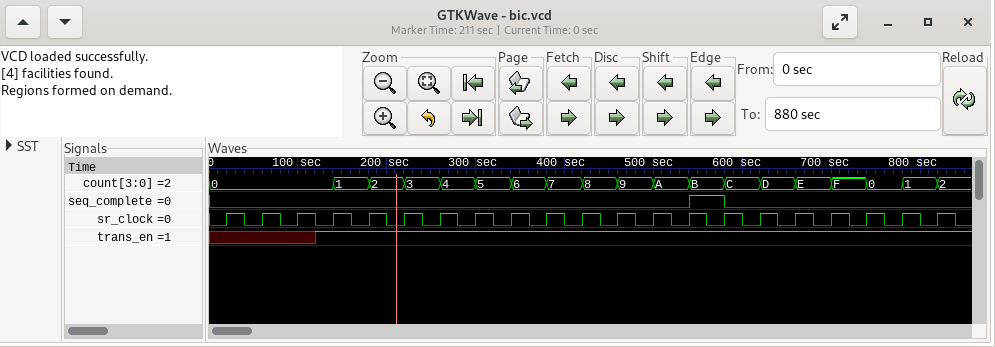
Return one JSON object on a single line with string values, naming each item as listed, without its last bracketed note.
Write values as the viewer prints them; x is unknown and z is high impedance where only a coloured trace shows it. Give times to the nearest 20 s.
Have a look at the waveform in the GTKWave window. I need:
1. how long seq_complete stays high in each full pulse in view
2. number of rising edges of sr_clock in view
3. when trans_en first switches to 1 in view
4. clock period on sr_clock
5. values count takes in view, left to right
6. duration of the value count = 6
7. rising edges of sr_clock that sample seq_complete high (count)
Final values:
{"how long seq_complete stays high in each full pulse in view": "40 s", "number of rising edges of sr_clock in view": "21", "when trans_en first switches to 1 in view": "120 s", "clock period on sr_clock": "40 s", "values count takes in view, left to right": "0, 1, 2, 3, 4, 5, 6, 7, 8, 9, A, B, C, D, E, F, 0, 1, 2", "duration of the value count = 6": "40 s", "rising edges of sr_clock that sample seq_complete high": "1"}
